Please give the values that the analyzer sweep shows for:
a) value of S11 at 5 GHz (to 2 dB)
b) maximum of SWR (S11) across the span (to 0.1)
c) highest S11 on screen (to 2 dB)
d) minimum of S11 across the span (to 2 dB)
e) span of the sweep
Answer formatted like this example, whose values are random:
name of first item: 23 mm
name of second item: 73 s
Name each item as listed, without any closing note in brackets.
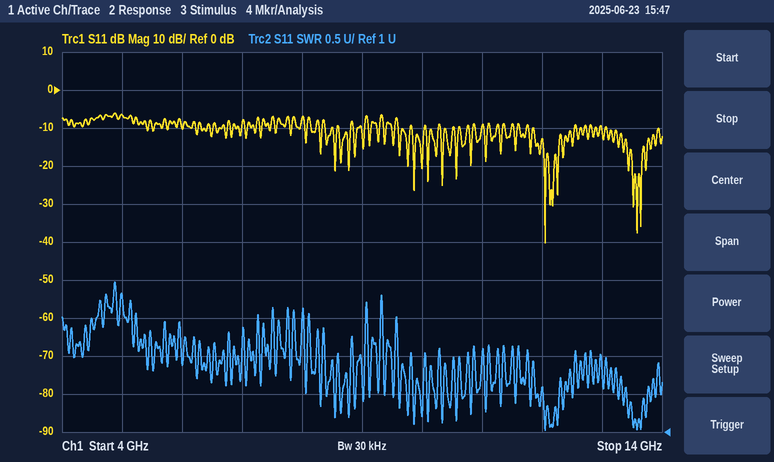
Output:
value of S11 at 5 GHz: -6 dB
maximum of SWR (S11) across the span: 3.0
highest S11 on screen: -6 dB
minimum of S11 across the span: -40 dB
span of the sweep: 10 GHz
